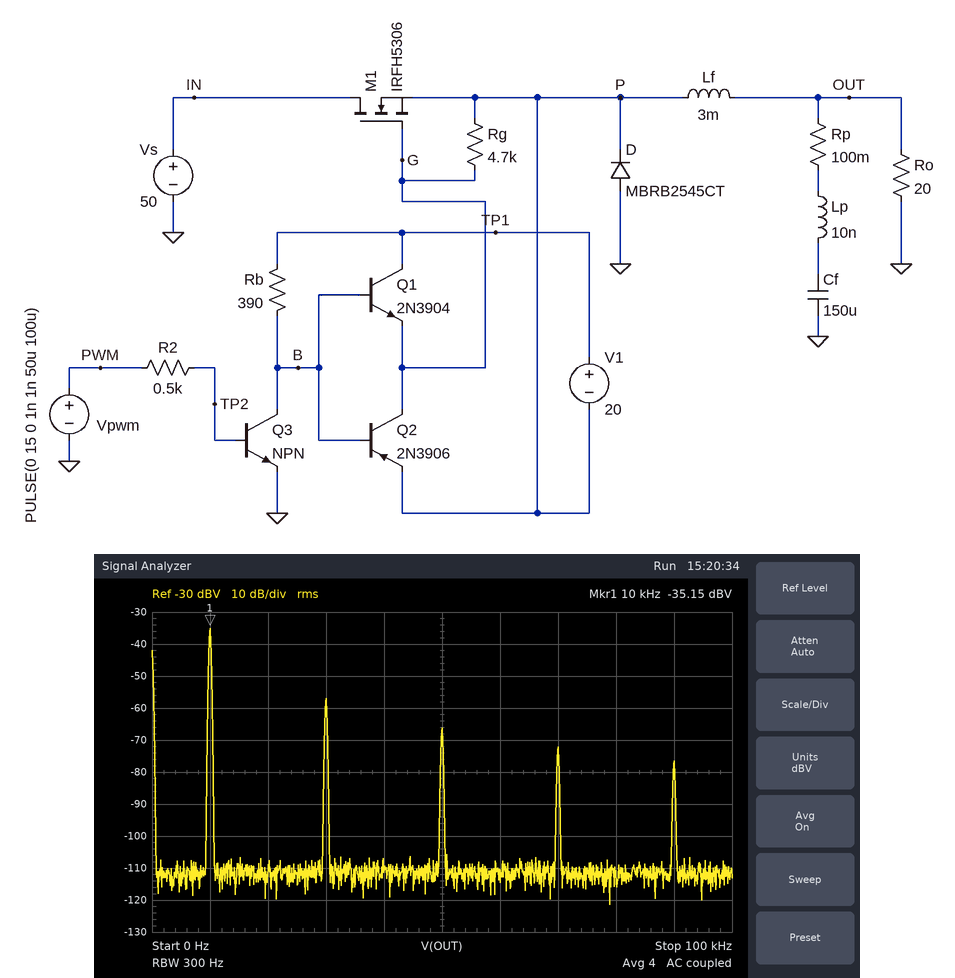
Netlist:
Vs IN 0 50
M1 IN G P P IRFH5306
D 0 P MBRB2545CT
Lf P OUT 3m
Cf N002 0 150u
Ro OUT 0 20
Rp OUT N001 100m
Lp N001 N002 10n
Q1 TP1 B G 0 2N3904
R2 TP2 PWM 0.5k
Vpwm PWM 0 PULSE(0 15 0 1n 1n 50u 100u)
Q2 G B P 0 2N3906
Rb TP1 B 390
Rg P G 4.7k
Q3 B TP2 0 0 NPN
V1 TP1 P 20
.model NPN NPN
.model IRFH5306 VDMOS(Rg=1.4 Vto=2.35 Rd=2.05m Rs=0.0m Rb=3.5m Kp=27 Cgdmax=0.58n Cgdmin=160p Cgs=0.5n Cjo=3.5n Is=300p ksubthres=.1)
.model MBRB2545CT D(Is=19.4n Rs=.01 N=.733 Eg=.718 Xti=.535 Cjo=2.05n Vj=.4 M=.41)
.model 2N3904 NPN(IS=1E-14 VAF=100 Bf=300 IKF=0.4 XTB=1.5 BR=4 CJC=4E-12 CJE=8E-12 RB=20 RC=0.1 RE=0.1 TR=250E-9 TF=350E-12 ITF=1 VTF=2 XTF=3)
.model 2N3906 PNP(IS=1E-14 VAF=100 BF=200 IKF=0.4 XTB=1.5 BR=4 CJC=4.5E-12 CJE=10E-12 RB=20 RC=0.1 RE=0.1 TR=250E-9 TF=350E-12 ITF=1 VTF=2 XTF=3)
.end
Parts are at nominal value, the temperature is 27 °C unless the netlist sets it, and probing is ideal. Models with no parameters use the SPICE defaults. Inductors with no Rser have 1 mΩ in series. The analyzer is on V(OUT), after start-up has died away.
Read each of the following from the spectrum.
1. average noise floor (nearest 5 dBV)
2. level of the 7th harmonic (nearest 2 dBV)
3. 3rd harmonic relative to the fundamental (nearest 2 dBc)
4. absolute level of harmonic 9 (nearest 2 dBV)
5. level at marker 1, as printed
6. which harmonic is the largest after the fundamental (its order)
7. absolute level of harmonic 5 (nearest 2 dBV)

-110 dBV
-72 dBV
-22 dBc
-76 dBV
-35.15 dBV
3
-66 dBV
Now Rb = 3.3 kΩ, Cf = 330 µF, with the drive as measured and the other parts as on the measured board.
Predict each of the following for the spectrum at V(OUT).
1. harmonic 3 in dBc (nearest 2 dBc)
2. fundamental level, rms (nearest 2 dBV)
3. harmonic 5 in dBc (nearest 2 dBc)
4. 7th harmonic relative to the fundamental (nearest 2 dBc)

-20 dBc
-38 dBV
-28 dBc
-34 dBc
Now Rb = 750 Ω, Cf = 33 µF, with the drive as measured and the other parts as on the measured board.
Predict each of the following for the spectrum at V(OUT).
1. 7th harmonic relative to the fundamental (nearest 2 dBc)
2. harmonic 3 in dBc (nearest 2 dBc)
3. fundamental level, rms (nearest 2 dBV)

-46 dBc
-28 dBc
-24 dBV
